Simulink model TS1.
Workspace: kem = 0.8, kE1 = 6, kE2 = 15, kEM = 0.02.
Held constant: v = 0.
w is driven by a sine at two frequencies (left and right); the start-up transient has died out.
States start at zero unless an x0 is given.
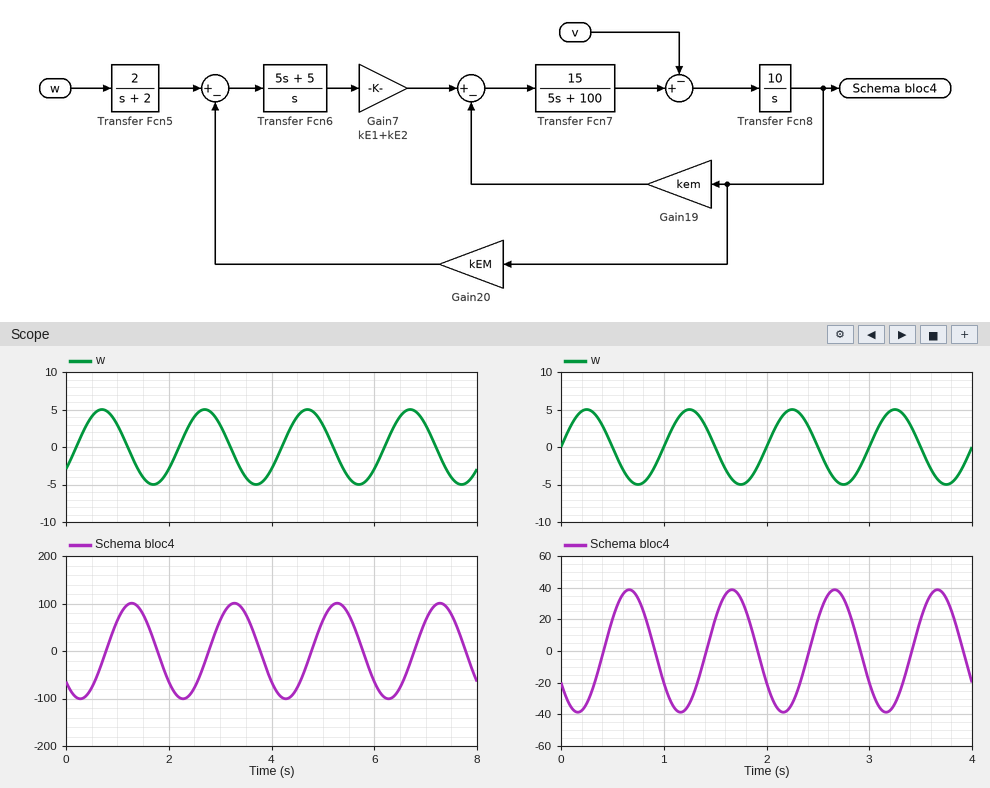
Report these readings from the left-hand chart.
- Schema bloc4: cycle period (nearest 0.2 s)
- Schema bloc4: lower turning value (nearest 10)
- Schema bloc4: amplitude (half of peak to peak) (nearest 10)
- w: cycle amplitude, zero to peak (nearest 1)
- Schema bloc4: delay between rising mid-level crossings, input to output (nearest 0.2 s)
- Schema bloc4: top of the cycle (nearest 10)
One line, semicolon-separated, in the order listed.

2.0 s; -100; 100; 5; 0.6 s; 100
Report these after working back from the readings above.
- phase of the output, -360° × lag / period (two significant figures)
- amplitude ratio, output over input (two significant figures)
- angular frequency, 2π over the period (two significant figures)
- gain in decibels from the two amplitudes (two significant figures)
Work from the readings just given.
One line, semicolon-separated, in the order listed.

-110°; 20; 3.1 rad/s; 26 dB
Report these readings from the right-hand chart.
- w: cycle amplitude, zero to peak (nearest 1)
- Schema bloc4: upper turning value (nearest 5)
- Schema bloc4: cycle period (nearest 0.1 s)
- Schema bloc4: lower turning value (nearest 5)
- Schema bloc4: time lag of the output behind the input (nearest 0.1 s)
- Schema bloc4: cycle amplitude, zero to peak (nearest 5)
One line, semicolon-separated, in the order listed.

5; 40; 1.0 s; -40; 0.4 s; 40
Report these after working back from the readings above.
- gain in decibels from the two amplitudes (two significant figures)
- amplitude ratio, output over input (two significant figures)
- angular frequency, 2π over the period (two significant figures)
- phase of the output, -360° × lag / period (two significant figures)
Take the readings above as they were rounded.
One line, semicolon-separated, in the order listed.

18 dB; 8.0; 6.3 rad/s; -140°
